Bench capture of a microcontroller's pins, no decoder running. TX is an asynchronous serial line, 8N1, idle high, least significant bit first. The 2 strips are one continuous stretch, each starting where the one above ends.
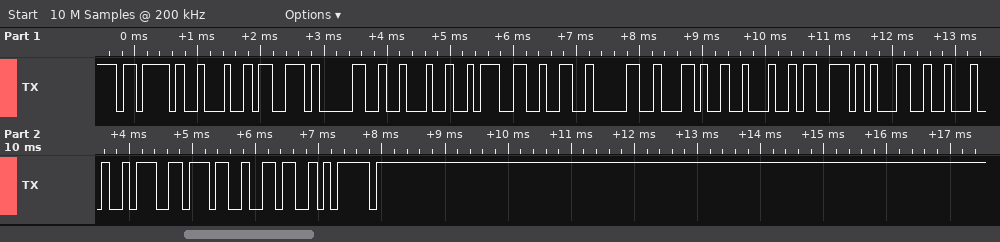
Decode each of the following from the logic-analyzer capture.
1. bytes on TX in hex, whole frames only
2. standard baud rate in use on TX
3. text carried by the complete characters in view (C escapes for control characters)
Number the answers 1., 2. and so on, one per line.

1. 0x7B 0x22 0x73 0x30 0x22 0x3A 0x32 0x30 0x2C 0x22 0x73 0x31 0x22 0x3A 0x37 0x36 0x7D
2. 9600 baud
3. "{\"s0\":20,\"s1\":76}"
